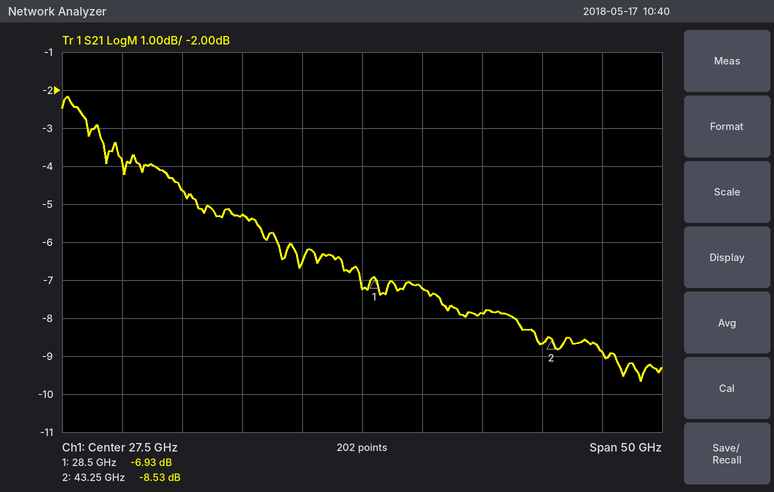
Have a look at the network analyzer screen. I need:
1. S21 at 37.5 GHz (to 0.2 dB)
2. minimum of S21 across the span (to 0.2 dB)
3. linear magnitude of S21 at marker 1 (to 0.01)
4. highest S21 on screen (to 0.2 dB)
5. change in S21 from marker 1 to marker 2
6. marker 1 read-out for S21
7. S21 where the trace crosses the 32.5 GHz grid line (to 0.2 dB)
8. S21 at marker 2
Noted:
-7.8 dB
-9.6 dB
0.45
-2.2 dB
-1.60 dB
-6.93 dB
-7.2 dB
-8.53 dB
